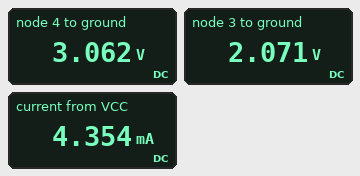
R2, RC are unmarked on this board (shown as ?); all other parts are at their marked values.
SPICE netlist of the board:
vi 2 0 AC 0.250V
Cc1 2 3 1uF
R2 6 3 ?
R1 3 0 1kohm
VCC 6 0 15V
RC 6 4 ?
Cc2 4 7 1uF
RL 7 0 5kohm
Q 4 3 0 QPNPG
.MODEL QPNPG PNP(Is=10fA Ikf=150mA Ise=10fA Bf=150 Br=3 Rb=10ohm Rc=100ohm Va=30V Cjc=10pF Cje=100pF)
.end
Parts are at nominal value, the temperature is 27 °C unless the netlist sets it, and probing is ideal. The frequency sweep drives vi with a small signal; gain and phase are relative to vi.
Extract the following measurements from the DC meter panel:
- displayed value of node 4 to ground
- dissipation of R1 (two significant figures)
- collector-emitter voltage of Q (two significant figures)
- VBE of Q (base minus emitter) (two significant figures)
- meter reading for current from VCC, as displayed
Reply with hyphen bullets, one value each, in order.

- 3.062 V
- 4.3 mW
- 3.1 V
- 2.1 V
- 4.354 mA
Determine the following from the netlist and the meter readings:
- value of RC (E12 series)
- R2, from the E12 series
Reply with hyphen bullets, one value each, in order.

- 3.9 kΩ
- 10 kΩ
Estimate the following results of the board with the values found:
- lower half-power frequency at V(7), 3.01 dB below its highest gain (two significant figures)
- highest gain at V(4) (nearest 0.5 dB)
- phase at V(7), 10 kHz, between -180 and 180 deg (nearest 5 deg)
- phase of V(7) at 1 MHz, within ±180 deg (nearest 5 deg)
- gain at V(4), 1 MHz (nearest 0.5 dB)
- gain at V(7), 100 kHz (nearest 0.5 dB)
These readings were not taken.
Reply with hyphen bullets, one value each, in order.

- 200 Hz
- -0.5 dB
- 0 deg
- 0 deg
- -0.5 dB
- -0.5 dB
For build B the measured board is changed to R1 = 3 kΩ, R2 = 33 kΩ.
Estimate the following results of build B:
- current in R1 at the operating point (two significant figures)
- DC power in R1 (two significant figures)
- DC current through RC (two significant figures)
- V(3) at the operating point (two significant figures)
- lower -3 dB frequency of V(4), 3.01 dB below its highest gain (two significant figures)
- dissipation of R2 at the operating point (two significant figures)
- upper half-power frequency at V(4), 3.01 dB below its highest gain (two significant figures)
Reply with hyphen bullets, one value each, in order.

- 1.1 mA
- 3.4 mW
- 2.8 mA
- 3.2 V
- 77 Hz
- 4.2 mW
- 280 MHz
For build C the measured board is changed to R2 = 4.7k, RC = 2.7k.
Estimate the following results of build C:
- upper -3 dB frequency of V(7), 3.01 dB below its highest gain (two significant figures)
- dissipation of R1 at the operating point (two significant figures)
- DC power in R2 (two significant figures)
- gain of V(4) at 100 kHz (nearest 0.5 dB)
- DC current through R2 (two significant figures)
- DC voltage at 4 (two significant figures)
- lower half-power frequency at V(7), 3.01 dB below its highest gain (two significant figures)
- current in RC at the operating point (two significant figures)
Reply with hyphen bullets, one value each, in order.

- 280 MHz
- 12 mW
- 28 mW
- -0.5 dB
- 2.5 mA
- 4.5 V
- 220 Hz
- 3.9 mA
